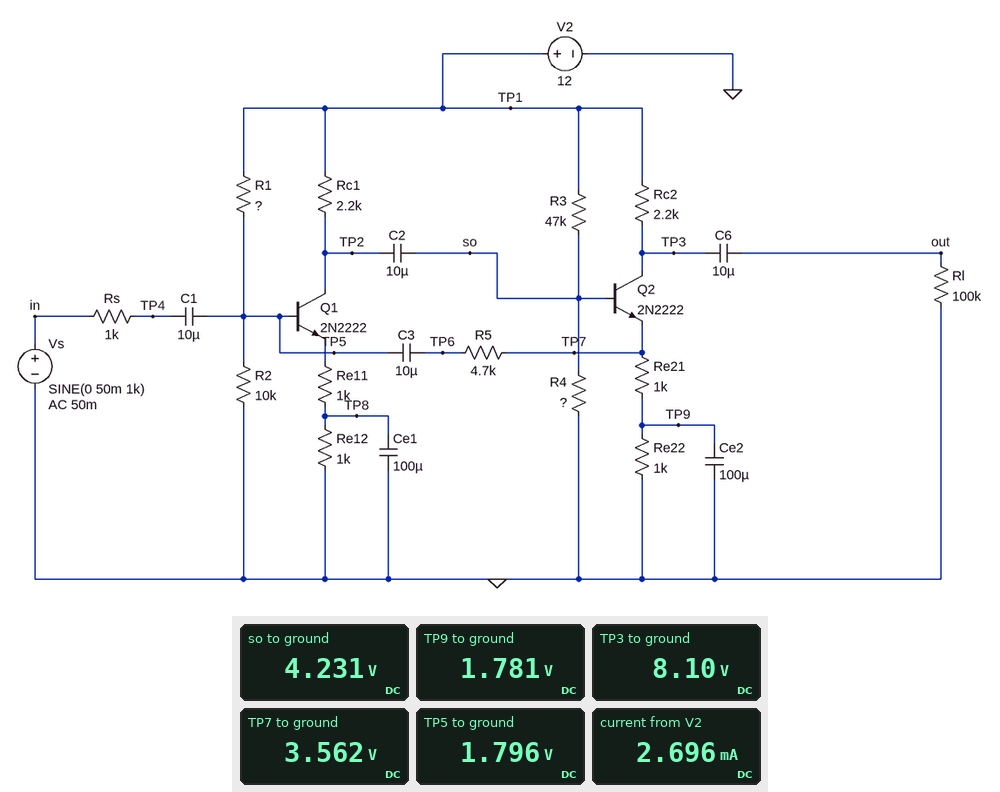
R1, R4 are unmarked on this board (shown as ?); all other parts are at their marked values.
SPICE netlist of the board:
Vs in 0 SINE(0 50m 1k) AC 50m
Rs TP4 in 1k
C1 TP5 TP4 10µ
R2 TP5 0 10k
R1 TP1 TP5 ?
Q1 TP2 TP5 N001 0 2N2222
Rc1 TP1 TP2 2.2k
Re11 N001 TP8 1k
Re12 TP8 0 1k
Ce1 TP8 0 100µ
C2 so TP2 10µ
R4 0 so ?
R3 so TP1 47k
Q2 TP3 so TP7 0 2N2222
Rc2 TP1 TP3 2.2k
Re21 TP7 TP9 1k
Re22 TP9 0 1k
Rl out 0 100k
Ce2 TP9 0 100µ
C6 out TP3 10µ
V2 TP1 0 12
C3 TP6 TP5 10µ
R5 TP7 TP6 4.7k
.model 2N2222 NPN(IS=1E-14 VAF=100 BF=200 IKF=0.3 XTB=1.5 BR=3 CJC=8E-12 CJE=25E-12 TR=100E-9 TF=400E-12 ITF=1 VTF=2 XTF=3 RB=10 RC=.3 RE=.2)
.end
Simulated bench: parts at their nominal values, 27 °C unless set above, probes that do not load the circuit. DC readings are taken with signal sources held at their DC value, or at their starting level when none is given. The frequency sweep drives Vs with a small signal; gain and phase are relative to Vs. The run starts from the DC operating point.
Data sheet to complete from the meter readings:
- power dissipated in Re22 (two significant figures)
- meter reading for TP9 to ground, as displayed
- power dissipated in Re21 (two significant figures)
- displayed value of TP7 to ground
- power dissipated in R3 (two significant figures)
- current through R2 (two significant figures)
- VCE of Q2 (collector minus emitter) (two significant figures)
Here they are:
3.2 mW
1.781 V
3.2 mW
3.562 V
1.3 mW
180 µA
4.5 V
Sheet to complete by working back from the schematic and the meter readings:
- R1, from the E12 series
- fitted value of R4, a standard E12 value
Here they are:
56 kΩ
27 kΩ
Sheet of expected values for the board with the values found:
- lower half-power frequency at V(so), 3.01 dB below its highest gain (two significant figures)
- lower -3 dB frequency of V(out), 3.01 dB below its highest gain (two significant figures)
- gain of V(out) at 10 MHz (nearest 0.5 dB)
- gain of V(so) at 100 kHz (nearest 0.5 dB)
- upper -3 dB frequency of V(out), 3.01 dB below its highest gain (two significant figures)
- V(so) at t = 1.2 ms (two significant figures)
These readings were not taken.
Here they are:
8.0 Hz
8.9 Hz
0.5 dB
0.5 dB
3.9 MHz
4.2 V
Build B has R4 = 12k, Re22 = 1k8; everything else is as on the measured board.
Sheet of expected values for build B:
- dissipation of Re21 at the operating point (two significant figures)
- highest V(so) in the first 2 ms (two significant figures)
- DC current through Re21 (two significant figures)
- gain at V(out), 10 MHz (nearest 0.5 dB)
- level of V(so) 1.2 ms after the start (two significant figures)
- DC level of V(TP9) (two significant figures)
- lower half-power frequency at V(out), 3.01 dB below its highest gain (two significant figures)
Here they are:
400 µW
2.5 V
630 µA
1.0 dB
2.4 V
1.1 V
8.6 Hz
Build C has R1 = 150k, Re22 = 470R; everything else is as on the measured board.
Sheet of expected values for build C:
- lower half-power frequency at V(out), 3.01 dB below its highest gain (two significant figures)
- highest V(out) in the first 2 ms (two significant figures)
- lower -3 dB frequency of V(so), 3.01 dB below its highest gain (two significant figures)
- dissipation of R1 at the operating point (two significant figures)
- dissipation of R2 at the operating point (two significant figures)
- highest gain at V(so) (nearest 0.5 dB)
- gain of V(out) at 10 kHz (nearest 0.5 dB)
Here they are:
8.7 Hz
130 mV
7.3 Hz
840 µW
56 µW
-1.0 dB
8.0 dB
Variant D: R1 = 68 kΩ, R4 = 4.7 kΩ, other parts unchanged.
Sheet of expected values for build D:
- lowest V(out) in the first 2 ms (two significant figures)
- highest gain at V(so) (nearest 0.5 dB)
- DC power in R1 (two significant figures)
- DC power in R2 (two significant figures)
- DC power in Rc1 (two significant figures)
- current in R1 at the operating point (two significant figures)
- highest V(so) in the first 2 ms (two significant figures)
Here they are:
-110 mV
-1.5 dB
1.6 mW
230 µW
430 µW
150 µA
1.1 V
